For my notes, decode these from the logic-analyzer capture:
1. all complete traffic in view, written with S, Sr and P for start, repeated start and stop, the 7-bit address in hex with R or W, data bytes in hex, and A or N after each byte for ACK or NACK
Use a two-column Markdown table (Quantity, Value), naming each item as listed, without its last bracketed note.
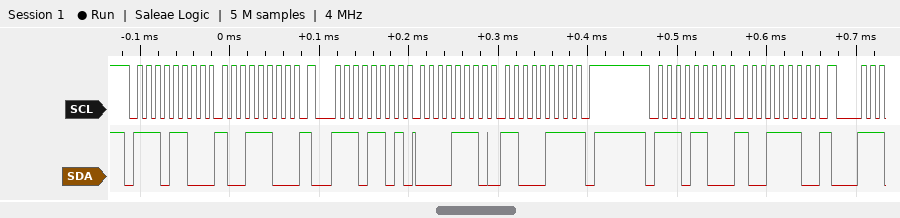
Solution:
| Quantity | Value |
|---|---|
| all complete traffic in view, written with S, Sr and P for start, repeated start and stop, the 7-bit address in hex with R or W, data bytes in hex, and A or N after each byte for ACK or NACK | S 76W A 9C A Sr 76R A 0E A C7 N P S 76W A 9E A |
